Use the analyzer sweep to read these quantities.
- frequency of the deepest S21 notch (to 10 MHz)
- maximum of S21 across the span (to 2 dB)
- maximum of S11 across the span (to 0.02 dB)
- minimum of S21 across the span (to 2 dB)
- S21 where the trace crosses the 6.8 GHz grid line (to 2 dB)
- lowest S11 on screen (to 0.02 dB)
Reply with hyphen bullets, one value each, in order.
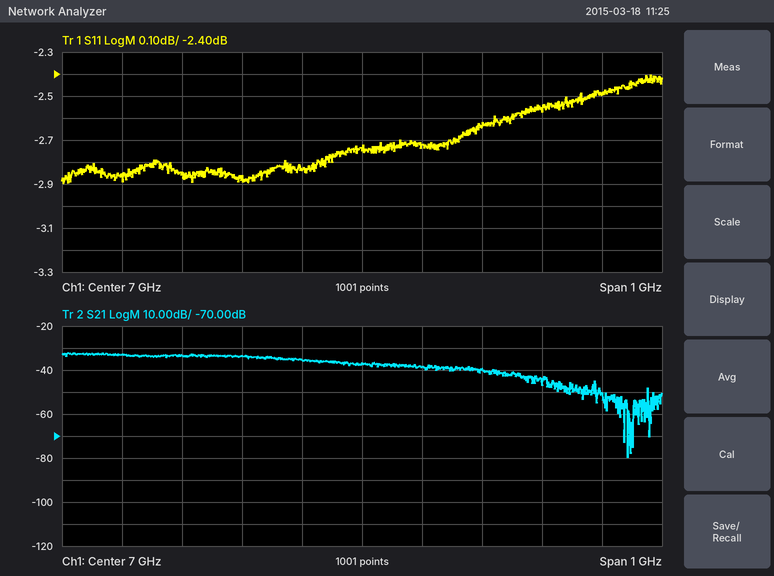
- 7.44 GHz
- -32 dB
- -2.40 dB
- -80 dB
- -34 dB
- -2.90 dB
